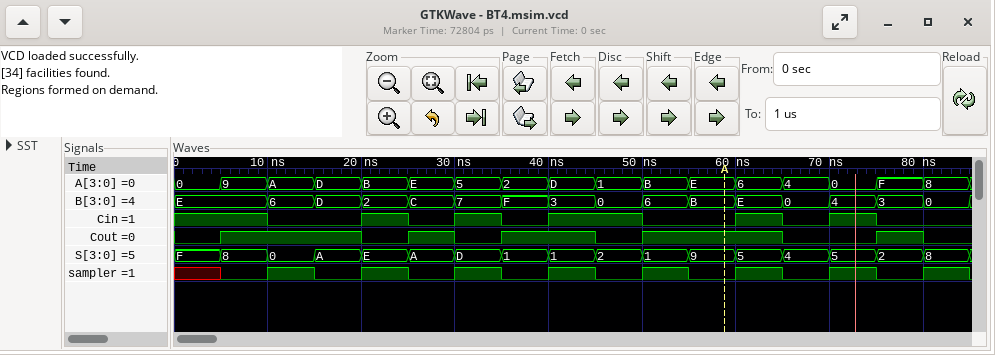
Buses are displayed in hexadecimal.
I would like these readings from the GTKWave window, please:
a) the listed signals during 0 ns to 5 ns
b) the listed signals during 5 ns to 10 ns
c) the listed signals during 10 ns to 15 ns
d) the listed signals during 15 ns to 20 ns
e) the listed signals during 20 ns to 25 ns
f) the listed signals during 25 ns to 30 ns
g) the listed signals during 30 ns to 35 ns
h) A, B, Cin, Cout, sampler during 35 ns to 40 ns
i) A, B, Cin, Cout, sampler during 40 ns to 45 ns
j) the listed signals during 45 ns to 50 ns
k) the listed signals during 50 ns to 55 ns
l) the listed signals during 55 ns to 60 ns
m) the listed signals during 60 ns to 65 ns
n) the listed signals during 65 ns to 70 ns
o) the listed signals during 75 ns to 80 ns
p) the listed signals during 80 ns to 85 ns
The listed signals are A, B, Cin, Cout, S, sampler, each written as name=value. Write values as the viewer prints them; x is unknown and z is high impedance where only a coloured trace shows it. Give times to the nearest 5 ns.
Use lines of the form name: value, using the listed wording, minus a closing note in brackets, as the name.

the listed signals during 0 ns to 5 ns: A=0, B=E, Cin=1, Cout=0, S=F, sampler=x
the listed signals during 5 ns to 10 ns: A=9, B=E, Cin=1, Cout=1, S=8, sampler=0
the listed signals during 10 ns to 15 ns: A=A, B=6, Cin=0, Cout=1, S=0, sampler=1
the listed signals during 15 ns to 20 ns: A=D, B=D, Cin=0, Cout=1, S=A, sampler=0
the listed signals during 20 ns to 25 ns: A=B, B=2, Cin=1, Cout=0, S=E, sampler=1
the listed signals during 25 ns to 30 ns: A=E, B=C, Cin=0, Cout=1, S=A, sampler=0
the listed signals during 30 ns to 35 ns: A=5, B=7, Cin=1, Cout=0, S=D, sampler=1
A, B, Cin, Cout, sampler during 35 ns to 40 ns: A=2, B=F, Cin=0, Cout=1, sampler=0
A, B, Cin, Cout, sampler during 40 ns to 45 ns: A=D, B=3, Cin=1, Cout=1, sampler=1
the listed signals during 45 ns to 50 ns: A=1, B=0, Cin=1, Cout=0, S=2, sampler=0
the listed signals during 50 ns to 55 ns: A=B, B=6, Cin=0, Cout=1, S=1, sampler=1
the listed signals during 55 ns to 60 ns: A=E, B=B, Cin=0, Cout=1, S=9, sampler=0
the listed signals during 60 ns to 65 ns: A=6, B=E, Cin=1, Cout=1, S=5, sampler=1
the listed signals during 65 ns to 70 ns: A=4, B=0, Cin=0, Cout=0, S=4, sampler=0
the listed signals during 75 ns to 80 ns: A=F, B=3, Cin=0, Cout=1, S=2, sampler=0
the listed signals during 80 ns to 85 ns: A=8, B=0, Cin=0, Cout=0, S=8, sampler=1
